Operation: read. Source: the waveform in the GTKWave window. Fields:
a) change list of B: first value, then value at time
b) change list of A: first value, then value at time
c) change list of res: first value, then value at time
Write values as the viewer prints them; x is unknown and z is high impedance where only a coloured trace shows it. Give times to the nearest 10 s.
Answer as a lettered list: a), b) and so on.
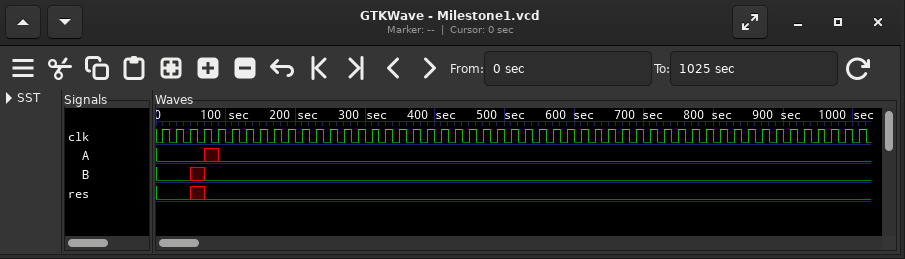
a) 0, x at 50 s, 0 at 70 s
b) 0, x at 70 s, 0 at 90 s
c) 0, x at 50 s, 0 at 70 s
